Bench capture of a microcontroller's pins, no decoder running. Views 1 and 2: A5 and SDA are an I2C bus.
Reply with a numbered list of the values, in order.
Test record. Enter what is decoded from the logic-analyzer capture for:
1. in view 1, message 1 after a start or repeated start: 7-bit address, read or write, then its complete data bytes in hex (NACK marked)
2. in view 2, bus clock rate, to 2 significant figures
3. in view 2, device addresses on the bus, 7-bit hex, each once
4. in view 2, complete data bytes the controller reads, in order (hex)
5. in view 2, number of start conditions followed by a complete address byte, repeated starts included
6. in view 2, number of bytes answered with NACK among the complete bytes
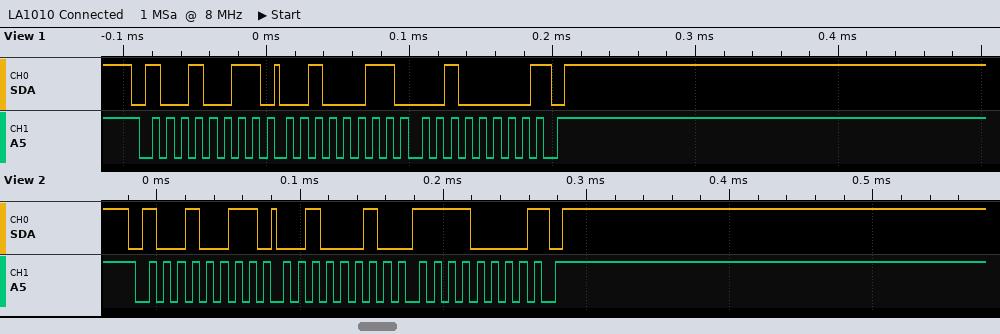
1. 0x49 read: 23 20 NACK
2. 100 kHz
3. 0x49
4. 22 F0
5. 1
6. 1
